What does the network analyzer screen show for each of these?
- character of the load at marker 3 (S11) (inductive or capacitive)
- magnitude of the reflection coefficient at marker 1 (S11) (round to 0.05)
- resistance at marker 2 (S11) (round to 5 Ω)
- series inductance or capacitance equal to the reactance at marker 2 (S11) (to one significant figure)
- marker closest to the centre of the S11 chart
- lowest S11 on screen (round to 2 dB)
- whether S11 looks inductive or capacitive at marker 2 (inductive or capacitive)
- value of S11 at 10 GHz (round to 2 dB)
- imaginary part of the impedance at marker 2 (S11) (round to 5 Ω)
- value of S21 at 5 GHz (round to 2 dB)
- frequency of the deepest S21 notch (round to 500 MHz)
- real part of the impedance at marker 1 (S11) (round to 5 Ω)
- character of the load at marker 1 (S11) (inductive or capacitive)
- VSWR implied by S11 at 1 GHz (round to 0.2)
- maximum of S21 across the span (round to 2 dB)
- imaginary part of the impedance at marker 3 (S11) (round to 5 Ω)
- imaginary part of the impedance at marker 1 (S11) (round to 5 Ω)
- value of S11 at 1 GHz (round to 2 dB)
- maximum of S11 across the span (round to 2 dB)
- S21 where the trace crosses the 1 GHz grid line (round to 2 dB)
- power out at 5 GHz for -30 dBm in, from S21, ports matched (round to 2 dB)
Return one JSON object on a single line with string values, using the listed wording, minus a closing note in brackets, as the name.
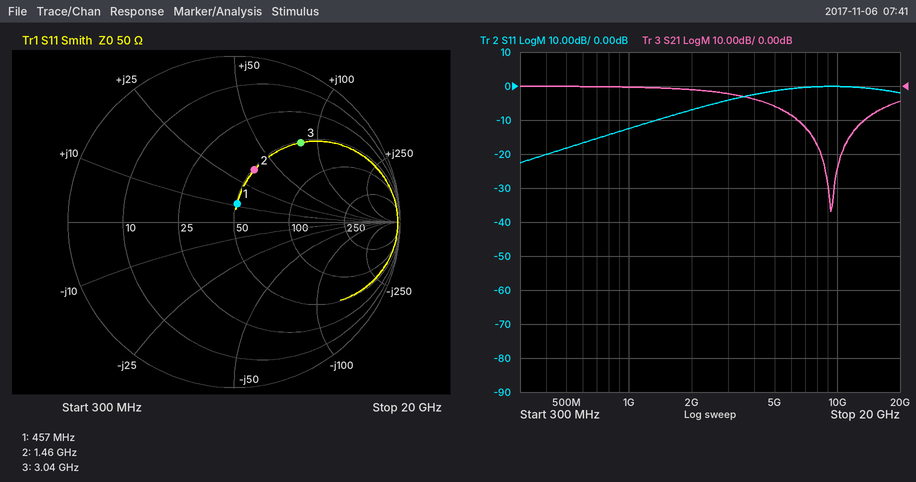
{"character of the load at marker 3 (S11)": "inductive", "magnitude of the reflection coefficient at marker 1 (S11)": "0.10", "resistance at marker 2 (S11)": "50 Ω", "series inductance or capacitance equal to the reactance at marker 2 (S11)": "4 nH", "marker closest to the centre of the S11 chart": "marker 1", "lowest S11 on screen": "-22 dB", "whether S11 looks inductive or capacitive at marker 2": "inductive", "value of S11 at 10 GHz": "0 dB", "imaginary part of the impedance at marker 2 (S11)": "+35 Ω", "value of S21 at 5 GHz": "-6 dB", "frequency of the deepest S21 notch": "9.5 GHz", "real part of the impedance at marker 1 (S11)": "50 Ω", "character of the load at marker 1 (S11)": "inductive", "VSWR implied by S11 at 1 GHz": "1.6", "maximum of S21 across the span": "0 dB", "imaginary part of the impedance at marker 3 (S11)": "+80 Ω", "imaginary part of the impedance at marker 1 (S11)": "+10 Ω", "value of S11 at 1 GHz": "-12 dB", "maximum of S11 across the span": "0 dB", "S21 where the trace crosses the 1 GHz grid line": "0 dB", "power out at 5 GHz for -30 dBm in, from S21, ports matched": "-36 dBm"}
